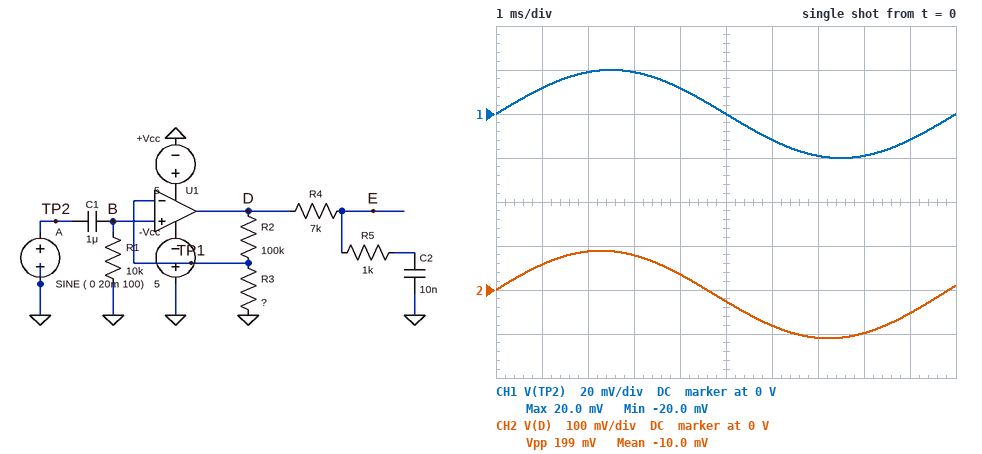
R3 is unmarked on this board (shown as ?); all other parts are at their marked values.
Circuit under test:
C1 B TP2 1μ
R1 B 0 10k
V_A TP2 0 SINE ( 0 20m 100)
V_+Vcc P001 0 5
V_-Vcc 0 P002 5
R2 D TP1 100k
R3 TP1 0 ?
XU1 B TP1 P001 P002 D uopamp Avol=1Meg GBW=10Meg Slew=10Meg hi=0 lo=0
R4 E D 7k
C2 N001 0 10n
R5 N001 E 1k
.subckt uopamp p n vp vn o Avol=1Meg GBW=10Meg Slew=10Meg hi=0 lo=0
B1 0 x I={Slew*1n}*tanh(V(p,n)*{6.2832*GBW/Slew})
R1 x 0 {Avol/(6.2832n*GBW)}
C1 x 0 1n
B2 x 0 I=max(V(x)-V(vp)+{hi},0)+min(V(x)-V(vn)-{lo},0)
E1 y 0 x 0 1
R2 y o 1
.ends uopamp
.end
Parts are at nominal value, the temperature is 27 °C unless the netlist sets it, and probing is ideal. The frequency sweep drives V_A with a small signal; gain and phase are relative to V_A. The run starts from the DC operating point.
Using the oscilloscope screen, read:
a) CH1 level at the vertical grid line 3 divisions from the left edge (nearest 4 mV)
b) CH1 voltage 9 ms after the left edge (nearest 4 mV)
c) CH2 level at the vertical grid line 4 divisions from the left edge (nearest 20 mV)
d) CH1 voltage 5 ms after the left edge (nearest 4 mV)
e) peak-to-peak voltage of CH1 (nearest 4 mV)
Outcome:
20 mV
-12 mV
40 mV
0 V
40 mV
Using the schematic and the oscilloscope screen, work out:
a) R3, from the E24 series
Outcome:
24 kΩ
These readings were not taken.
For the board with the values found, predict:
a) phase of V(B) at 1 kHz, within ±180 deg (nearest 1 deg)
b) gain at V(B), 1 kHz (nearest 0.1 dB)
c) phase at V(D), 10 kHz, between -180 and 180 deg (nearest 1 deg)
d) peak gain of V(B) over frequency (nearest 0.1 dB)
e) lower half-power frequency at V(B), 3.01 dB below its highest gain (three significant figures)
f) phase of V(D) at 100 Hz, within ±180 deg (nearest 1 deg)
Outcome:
1 deg
0 dB
0 deg
0 dB
15.9 Hz
9 deg
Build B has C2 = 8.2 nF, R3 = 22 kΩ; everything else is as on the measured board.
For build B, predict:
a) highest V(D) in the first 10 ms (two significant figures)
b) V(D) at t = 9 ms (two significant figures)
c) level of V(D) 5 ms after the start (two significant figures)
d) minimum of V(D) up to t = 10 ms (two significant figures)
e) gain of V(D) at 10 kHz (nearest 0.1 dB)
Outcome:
96 mV
-57 mV
-28 mV
-120 mV
14.9 dB
